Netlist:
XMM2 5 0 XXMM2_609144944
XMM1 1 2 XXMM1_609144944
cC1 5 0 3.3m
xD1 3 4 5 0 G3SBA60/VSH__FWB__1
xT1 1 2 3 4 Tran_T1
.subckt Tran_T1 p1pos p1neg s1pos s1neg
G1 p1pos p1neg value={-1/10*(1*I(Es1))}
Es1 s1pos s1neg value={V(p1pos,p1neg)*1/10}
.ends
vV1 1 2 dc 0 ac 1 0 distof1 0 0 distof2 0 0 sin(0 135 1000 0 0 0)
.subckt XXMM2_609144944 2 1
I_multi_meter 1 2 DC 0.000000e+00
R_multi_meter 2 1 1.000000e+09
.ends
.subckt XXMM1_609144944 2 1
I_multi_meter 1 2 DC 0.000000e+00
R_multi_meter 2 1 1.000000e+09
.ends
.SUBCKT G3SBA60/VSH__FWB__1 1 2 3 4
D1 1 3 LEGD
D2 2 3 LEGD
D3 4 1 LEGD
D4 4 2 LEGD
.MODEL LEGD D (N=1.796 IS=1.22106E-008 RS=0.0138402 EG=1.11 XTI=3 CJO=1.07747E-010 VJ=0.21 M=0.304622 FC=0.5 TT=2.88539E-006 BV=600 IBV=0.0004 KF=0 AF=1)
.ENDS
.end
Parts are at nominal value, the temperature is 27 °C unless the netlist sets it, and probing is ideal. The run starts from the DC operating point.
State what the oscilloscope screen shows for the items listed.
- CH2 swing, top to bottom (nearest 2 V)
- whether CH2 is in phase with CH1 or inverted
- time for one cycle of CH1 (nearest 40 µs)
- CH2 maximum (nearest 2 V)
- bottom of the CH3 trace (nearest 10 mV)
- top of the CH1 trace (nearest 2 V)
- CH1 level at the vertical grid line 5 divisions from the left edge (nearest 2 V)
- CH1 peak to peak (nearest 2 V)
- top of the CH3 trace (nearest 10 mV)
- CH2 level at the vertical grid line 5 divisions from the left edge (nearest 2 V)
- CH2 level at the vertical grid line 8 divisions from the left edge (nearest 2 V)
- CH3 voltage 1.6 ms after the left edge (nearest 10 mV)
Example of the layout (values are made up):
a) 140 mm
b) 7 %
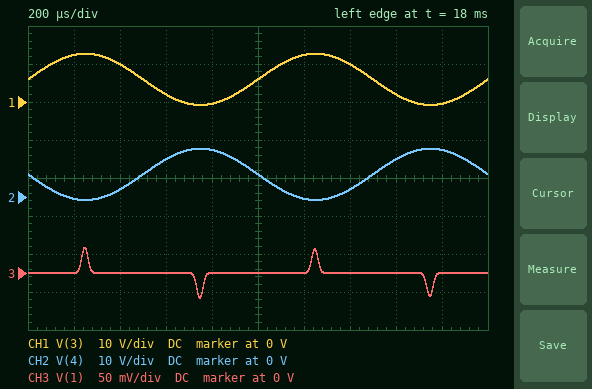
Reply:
a) 14 V
b) inverted
c) 1.00 ms
d) 12 V
e) -30 mV
f) 12 V
g) 6 V
h) 14 V
i) 30 mV
j) 6 V
k) 10 V
l) 0 V
